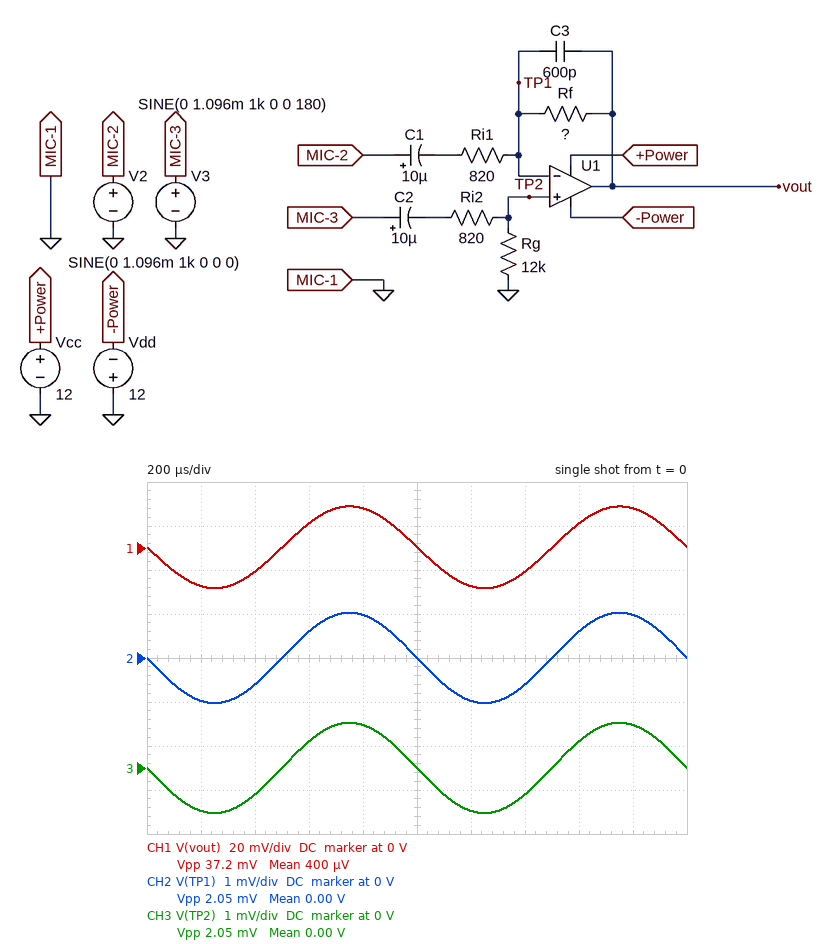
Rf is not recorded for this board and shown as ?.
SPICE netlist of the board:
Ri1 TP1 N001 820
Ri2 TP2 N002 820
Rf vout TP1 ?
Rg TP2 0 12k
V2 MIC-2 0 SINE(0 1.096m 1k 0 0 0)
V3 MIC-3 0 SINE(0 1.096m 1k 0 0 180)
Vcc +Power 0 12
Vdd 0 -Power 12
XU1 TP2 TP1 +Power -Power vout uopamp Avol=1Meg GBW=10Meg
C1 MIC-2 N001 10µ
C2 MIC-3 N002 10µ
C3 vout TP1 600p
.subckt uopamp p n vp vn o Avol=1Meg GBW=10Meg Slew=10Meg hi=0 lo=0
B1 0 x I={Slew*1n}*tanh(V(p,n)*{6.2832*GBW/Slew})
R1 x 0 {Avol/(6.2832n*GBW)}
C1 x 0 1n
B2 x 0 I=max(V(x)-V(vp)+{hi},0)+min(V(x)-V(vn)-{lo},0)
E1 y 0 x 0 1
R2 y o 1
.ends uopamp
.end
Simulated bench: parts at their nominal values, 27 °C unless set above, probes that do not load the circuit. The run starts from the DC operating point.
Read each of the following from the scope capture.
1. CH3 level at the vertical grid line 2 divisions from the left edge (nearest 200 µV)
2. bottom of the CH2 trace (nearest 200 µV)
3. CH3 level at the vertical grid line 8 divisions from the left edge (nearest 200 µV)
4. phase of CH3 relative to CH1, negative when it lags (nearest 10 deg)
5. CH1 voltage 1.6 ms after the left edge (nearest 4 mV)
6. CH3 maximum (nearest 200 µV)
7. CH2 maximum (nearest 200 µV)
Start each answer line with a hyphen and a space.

- -600 µV
- -1.0 mV
- 600 µV
- 0 deg
- 12 mV
- 1.0 mV
- 1.0 mV
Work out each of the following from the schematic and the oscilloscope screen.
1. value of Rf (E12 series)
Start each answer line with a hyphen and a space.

- 6.8 kΩ
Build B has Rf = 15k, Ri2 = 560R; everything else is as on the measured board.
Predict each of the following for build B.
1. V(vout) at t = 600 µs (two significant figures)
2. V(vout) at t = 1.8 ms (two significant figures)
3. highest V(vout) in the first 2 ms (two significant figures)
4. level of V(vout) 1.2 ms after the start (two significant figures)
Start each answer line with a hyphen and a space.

- 23 mV
- 39 mV
- 41 mV
- -37 mV
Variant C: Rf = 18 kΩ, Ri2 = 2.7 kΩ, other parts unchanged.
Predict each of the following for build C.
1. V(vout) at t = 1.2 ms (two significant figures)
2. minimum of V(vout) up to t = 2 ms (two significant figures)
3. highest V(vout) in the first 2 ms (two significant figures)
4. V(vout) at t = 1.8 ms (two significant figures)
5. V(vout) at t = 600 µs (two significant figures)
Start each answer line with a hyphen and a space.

- -41 mV
- -44 mV
- 45 mV
- 44 mV
- 25 mV
